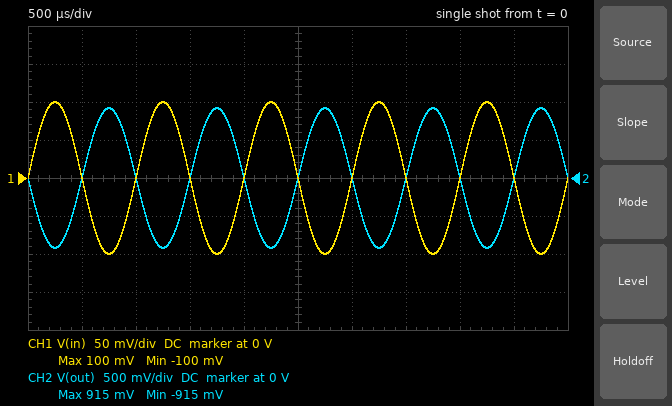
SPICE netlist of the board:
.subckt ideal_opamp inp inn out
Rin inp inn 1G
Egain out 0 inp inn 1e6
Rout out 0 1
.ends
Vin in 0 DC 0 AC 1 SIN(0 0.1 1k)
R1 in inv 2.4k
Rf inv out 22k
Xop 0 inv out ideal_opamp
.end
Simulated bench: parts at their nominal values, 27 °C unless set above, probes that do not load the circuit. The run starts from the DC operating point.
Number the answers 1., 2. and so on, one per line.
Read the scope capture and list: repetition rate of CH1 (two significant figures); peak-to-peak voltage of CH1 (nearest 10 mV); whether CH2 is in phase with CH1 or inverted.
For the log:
1. 1.0 kHz
2. 200 mV
3. inverted
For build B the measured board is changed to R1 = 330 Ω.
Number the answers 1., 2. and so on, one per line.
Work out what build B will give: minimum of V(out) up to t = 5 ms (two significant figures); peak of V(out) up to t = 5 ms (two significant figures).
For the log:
1. -6.7 V
2. 6.7 V
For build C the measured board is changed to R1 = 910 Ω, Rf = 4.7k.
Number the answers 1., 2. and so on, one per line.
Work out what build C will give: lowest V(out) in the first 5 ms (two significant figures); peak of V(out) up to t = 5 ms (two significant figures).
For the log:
1. -520 mV
2. 520 mV
